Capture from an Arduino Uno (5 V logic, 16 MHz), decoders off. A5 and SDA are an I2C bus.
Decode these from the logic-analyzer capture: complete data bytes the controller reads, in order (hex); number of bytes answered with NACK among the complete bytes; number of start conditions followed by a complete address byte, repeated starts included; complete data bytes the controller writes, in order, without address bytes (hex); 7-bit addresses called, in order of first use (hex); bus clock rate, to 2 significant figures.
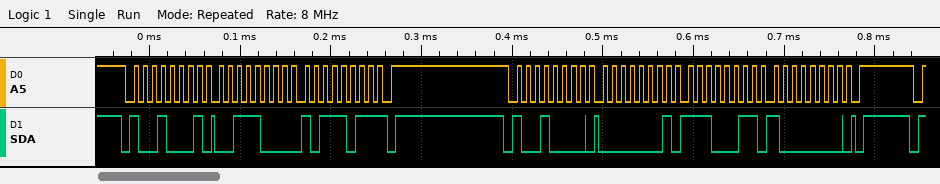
38 BB
1
2
01 E3 80
0x48
100 kHz
